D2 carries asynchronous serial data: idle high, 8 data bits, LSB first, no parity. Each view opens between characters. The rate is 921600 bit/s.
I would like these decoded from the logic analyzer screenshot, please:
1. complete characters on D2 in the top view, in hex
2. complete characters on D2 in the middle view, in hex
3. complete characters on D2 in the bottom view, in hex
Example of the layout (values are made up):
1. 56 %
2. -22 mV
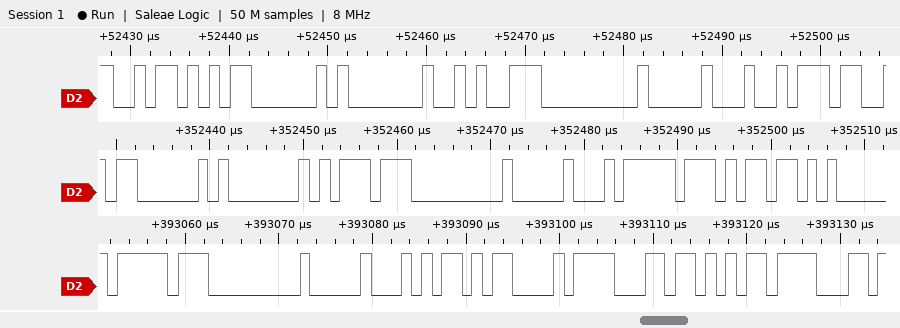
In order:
1. 5A, 03, 01, CA, 00, 10, BA
2. 03, 01, DD, 00, 10, DF, 6D
3. DF, 00, 10, AD, E8, 6C, ED
